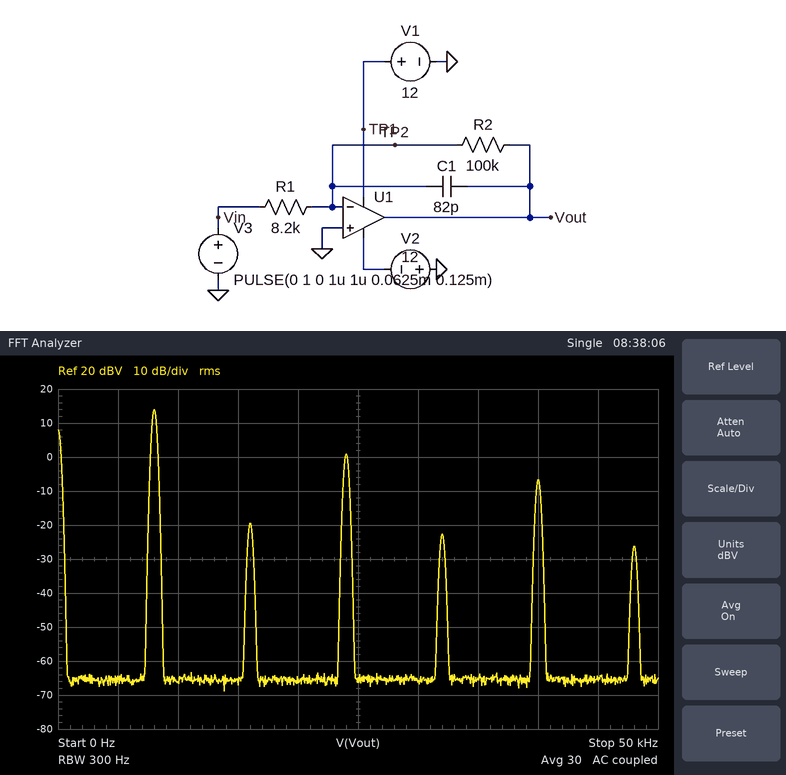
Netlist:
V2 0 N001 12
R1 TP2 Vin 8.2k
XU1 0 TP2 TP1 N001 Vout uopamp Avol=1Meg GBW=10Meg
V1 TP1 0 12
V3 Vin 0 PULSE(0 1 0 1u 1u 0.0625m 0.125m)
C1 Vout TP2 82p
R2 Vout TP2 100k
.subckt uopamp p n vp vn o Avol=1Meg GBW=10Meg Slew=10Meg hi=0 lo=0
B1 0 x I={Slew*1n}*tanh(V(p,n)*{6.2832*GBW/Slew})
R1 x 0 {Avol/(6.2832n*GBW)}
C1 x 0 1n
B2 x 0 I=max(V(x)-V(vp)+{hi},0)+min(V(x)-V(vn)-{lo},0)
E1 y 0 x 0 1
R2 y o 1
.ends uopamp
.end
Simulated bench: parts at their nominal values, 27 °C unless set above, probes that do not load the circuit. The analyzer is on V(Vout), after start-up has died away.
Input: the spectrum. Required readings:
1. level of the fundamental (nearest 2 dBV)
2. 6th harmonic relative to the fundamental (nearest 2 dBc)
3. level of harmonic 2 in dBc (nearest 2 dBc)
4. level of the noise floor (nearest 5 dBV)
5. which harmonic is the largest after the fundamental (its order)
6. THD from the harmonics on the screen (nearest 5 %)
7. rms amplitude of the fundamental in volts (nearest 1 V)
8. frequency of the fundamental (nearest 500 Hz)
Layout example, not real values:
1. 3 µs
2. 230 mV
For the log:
1. 14 dBV
2. -40 dBc
3. -34 dBc
4. -65 dBV
5. 3
6. 25 %
7. 5 V
8. 8.0 kHz
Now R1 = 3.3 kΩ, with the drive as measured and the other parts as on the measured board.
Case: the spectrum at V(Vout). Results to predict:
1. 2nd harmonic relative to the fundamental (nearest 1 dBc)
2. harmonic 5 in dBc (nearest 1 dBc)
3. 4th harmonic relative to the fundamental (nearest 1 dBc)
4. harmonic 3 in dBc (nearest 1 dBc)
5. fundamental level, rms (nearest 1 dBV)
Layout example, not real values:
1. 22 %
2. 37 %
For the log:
1. -16 dBc
2. -18 dBc
3. -20 dBc
4. -12 dBc
5. 14 dBV
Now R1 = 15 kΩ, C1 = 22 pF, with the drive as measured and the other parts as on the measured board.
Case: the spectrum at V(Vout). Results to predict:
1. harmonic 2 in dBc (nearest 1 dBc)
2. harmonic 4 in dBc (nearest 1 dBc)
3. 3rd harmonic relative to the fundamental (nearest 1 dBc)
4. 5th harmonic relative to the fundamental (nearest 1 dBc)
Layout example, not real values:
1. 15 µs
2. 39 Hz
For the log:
1. -32 dBc
2. -33 dBc
3. -10 dBc
4. -15 dBc
